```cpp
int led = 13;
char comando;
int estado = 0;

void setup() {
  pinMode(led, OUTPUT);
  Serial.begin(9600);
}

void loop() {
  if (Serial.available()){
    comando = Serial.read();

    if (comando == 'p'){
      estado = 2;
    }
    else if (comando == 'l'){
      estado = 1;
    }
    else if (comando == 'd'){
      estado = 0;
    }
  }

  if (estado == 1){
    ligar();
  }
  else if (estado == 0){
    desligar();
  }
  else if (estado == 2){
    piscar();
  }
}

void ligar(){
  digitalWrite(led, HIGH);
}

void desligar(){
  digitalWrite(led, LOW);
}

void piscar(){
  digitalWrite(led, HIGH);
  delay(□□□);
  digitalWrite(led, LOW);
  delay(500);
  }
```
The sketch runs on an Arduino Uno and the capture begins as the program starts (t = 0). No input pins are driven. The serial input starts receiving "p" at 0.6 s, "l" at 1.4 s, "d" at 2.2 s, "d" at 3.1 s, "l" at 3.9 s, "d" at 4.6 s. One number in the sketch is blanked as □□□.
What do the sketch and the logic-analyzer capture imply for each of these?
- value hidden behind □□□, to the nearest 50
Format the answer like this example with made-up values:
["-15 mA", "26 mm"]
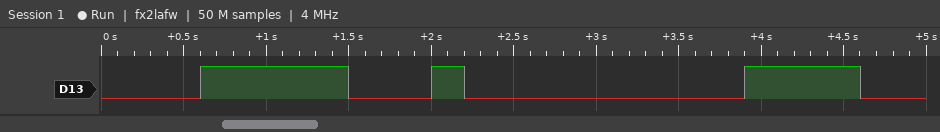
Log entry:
["900"]
